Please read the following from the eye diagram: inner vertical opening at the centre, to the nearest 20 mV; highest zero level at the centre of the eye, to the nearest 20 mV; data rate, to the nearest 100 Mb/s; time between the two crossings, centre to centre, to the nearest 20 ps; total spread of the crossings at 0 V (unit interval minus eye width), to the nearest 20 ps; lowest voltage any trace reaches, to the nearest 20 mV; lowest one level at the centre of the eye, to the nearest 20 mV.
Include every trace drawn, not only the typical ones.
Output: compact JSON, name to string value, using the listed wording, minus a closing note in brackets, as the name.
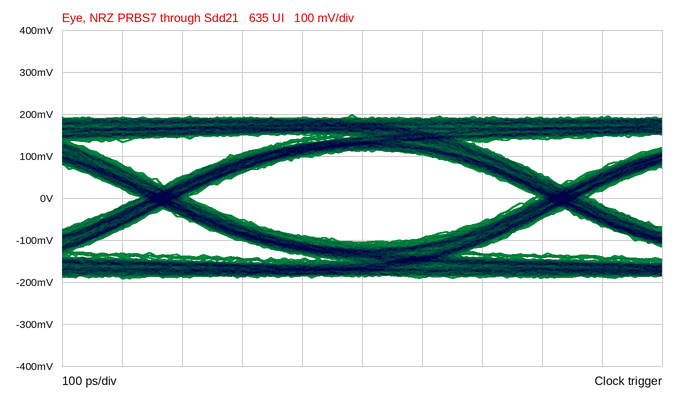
{"inner vertical opening at the centre, to the nearest 20 mV": "220 mV", "highest zero level at the centre of the eye, to the nearest 20 mV": "-100 mV", "data rate, to the nearest 100 Mb/s": "1.5 Gb/s", "time between the two crossings, centre to centre, to the nearest 20 ps": "660 ps", "total spread of the crossings at 0 V (unit interval minus eye width), to the nearest 20 ps": "100 ps", "lowest voltage any trace reaches, to the nearest 20 mV": "-200 mV", "lowest one level at the centre of the eye, to the nearest 20 mV": "120 mV"}
